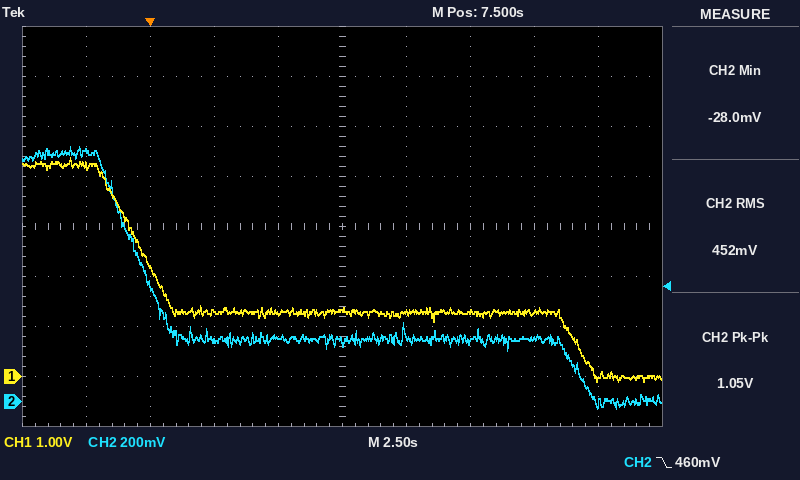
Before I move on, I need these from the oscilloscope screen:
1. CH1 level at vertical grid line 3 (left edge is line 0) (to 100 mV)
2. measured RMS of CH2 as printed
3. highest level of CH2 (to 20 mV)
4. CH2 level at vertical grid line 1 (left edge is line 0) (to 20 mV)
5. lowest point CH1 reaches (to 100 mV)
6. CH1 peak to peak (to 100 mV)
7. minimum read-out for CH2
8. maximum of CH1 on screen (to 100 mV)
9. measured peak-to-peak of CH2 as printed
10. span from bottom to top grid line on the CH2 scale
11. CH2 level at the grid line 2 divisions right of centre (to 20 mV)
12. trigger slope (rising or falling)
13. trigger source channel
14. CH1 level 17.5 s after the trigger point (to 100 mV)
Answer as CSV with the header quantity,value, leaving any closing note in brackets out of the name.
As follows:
quantity,value
CH1 level at vertical grid line 3 (left edge is line 0),1.3 V
measured RMS of CH2 as printed,452 mV
highest level of CH2,1.02 V
CH2 level at vertical grid line 1 (left edge is line 0),1.00 V
lowest point CH1 reaches,-100 mV
CH1 peak to peak,4.5 V
minimum read-out for CH2,-28.0 mV
maximum of CH1 on screen,4.4 V
measured peak-to-peak of CH2 as printed,1.05 V
span from bottom to top grid line on the CH2 scale,1.6 V
CH2 level at the grid line 2 divisions right of centre,240 mV
trigger slope,falling
trigger source channel,CH2
CH1 level 17.5 s after the trigger point,0.0 V
